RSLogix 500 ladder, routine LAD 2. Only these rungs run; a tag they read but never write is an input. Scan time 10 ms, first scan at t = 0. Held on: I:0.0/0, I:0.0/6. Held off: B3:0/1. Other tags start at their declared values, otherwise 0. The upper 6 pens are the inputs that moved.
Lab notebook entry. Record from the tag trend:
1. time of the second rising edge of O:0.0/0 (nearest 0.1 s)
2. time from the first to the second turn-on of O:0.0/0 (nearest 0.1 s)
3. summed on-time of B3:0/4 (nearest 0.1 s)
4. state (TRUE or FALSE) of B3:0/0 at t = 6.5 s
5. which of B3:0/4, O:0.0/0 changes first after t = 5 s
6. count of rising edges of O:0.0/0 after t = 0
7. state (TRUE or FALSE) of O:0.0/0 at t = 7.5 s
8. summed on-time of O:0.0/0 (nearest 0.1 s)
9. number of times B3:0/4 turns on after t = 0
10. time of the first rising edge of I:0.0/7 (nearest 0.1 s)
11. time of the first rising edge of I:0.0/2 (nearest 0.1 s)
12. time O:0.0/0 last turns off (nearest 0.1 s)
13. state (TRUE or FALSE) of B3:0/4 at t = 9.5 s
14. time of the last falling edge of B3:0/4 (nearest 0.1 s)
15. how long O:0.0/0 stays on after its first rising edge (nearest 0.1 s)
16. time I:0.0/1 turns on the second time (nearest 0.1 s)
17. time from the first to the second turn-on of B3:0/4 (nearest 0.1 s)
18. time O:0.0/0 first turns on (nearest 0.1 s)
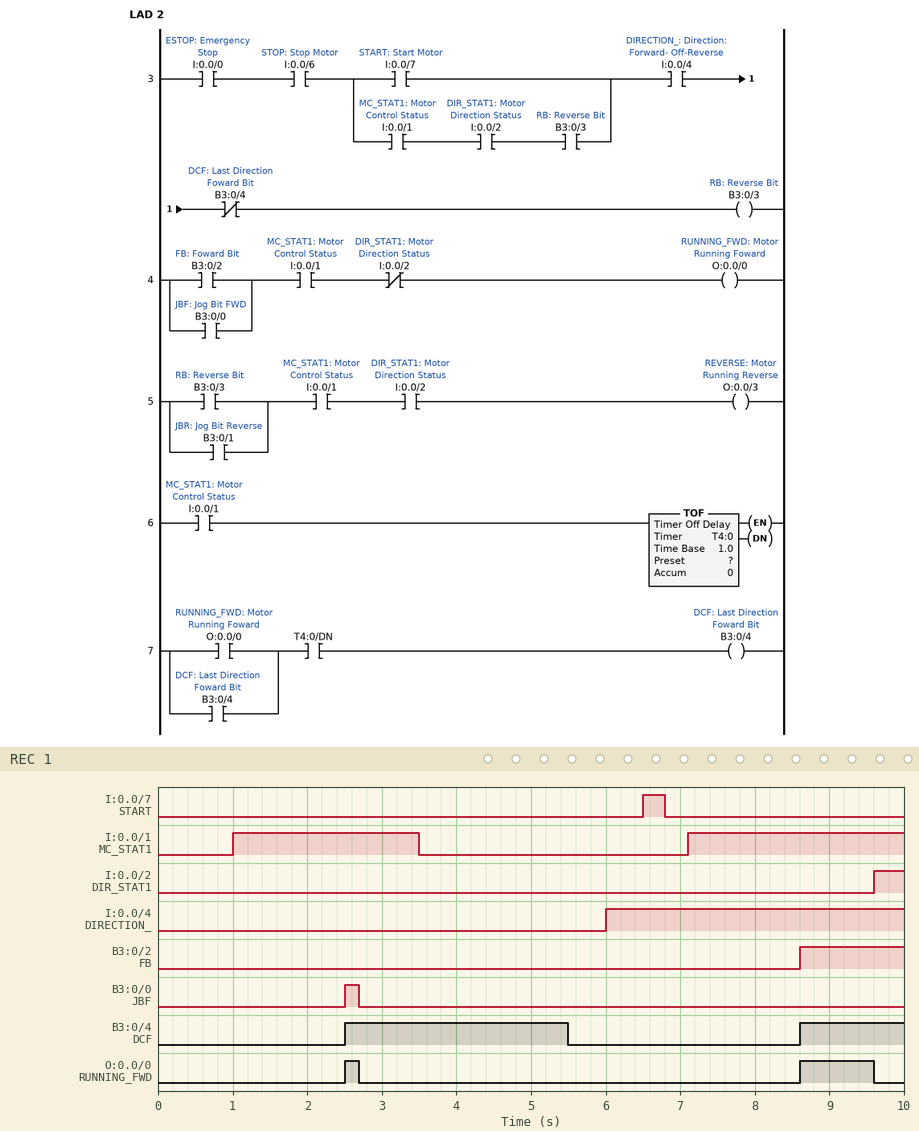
8.6 s
6.1 s
4.4 s
FALSE
B3:0/4
2
FALSE
1.2 s
2
6.5 s
9.6 s
9.6 s
TRUE
5.5 s
0.2 s
7.1 s
6.1 s
2.5 s
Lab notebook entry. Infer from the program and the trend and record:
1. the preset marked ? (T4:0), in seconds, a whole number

2 s
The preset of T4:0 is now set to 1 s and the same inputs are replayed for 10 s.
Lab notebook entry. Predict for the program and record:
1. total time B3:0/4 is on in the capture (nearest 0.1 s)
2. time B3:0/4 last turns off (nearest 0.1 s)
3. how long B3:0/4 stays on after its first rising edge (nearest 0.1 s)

3.4 s
4.5 s
2.0 s
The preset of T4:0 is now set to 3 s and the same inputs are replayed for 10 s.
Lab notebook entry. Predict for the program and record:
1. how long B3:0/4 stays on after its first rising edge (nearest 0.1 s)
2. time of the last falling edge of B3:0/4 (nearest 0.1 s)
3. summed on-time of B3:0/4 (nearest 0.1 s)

4.0 s
6.5 s
5.4 s
